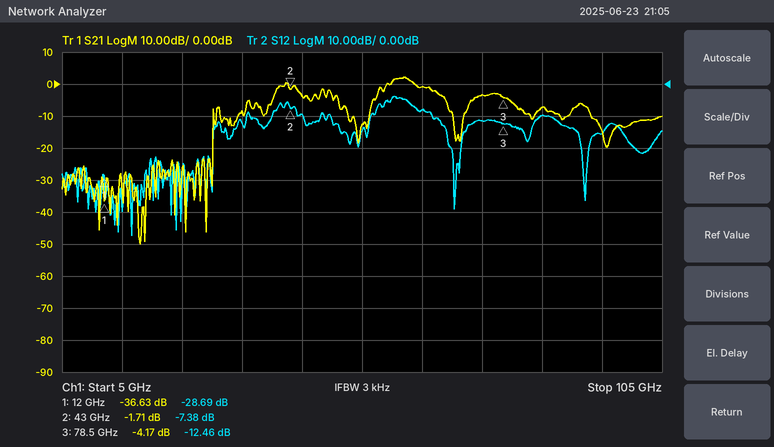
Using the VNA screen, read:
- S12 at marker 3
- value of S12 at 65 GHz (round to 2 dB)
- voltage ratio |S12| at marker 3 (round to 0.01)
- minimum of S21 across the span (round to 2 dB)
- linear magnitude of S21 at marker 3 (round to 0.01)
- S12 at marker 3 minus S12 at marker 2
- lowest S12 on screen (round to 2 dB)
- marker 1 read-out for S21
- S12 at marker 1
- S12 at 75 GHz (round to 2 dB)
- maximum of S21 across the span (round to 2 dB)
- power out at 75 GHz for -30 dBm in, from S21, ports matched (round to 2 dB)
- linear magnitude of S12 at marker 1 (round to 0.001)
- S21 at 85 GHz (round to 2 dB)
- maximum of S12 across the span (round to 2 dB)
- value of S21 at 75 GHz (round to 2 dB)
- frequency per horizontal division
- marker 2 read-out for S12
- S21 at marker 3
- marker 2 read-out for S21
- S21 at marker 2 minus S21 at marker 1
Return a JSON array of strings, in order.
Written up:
["-12.46 dB", "-8 dB", "0.24", "-50 dB", "0.62", "-5.08 dB", "-48 dB", "-36.63 dB", "-28.69 dB", "-12 dB", "2 dB", "-34 dBm", "0.037", "-8 dB", "-4 dB", "-4 dB", "10 GHz", "-7.38 dB", "-4.17 dB", "-1.71 dB", "34.92 dB"]
